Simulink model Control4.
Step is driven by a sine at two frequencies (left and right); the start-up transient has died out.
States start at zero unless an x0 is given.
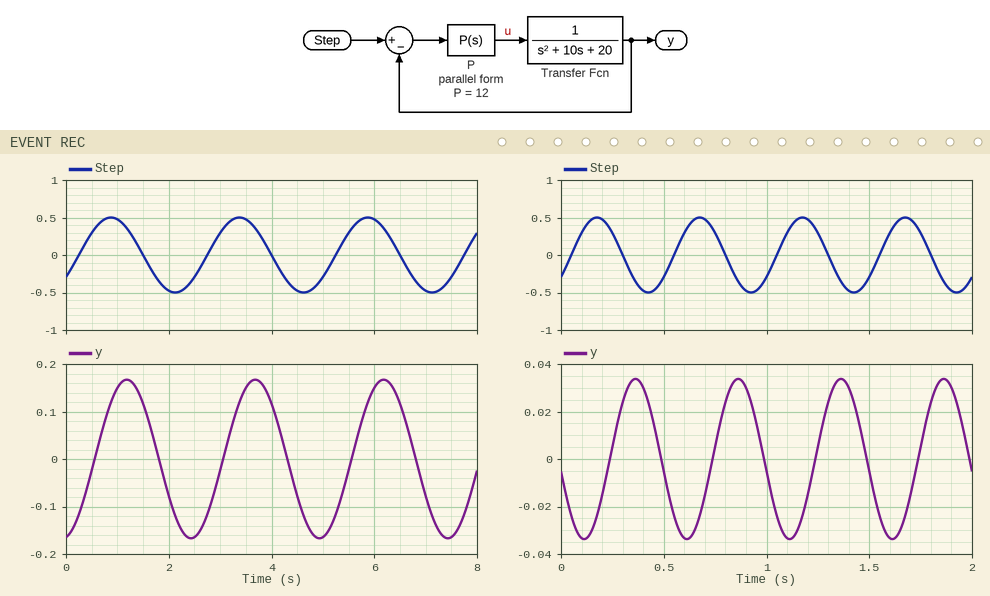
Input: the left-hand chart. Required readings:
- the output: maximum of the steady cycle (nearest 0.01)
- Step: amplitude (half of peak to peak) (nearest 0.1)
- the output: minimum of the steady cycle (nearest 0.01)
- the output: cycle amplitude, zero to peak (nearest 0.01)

0.17
0.5
-0.17
0.17
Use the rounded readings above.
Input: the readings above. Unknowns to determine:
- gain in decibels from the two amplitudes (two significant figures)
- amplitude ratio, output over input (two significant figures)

-9.4 dB
0.34
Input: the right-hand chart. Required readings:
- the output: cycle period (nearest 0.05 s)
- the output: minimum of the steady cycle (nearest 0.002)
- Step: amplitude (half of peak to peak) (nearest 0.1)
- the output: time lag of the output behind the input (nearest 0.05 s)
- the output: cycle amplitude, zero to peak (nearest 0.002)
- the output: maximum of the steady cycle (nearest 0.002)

0.50 s
-0.034
0.5
0.20 s
0.034
0.034
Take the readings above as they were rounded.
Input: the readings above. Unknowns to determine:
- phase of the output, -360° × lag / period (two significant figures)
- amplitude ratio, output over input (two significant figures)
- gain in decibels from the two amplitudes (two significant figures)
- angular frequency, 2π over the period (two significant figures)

-140°
0.068
-23 dB
13 rad/s
